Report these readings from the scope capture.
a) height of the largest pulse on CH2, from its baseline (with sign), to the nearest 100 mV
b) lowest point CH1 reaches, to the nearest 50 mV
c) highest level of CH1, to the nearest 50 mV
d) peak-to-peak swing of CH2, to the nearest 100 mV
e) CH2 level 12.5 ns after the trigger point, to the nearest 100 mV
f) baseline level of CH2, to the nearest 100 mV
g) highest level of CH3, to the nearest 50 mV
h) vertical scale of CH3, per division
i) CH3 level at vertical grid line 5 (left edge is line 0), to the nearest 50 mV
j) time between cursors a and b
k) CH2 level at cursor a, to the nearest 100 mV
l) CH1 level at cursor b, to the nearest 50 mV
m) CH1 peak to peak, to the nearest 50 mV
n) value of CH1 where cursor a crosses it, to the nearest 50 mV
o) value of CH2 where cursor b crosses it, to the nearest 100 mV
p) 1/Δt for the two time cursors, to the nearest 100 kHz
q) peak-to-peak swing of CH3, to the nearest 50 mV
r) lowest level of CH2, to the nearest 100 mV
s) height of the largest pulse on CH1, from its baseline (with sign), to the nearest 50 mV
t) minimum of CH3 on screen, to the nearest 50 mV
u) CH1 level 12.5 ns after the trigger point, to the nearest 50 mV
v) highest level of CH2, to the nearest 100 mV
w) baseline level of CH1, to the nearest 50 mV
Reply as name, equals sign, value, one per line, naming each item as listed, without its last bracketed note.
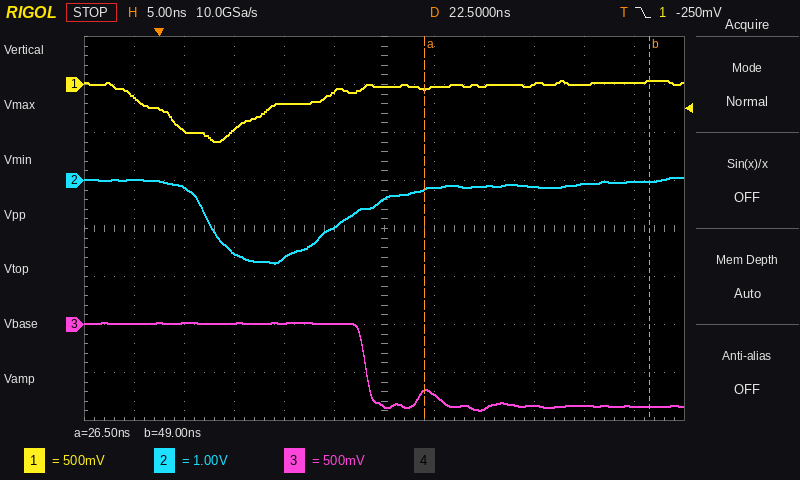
height of the largest pulse on CH2, from its baseline (with sign), to the nearest 100 mV = -1.6 V
lowest point CH1 reaches, to the nearest 50 mV = -600 mV
highest level of CH1, to the nearest 50 mV = 50 mV
peak-to-peak swing of CH2, to the nearest 100 mV = 1.8 V
CH2 level 12.5 ns after the trigger point, to the nearest 100 mV = -1.6 V
baseline level of CH2, to the nearest 100 mV = -100 mV
highest level of CH3, to the nearest 50 mV = 0 mV
vertical scale of CH3, per division = 500 mV
CH3 level at vertical grid line 5 (left edge is line 0), to the nearest 50 mV = 0 mV
time between cursors a and b = 22.5 ns
CH2 level at cursor a, to the nearest 100 mV = -200 mV
CH1 level at cursor b, to the nearest 50 mV = 50 mV
CH1 peak to peak, to the nearest 50 mV = 650 mV
value of CH1 where cursor a crosses it, to the nearest 50 mV = -50 mV
value of CH2 where cursor b crosses it, to the nearest 100 mV = 0.0 V
1/Δt for the two time cursors, to the nearest 100 kHz = 44.4 MHz
peak-to-peak swing of CH3, to the nearest 50 mV = 900 mV
lowest level of CH2, to the nearest 100 mV = -1.7 V
height of the largest pulse on CH1, from its baseline (with sign), to the nearest 50 mV = -600 mV
minimum of CH3 on screen, to the nearest 50 mV = -900 mV
CH1 level 12.5 ns after the trigger point, to the nearest 50 mV = -200 mV
highest level of CH2, to the nearest 100 mV = 100 mV
baseline level of CH1, to the nearest 50 mV = 0 mV
